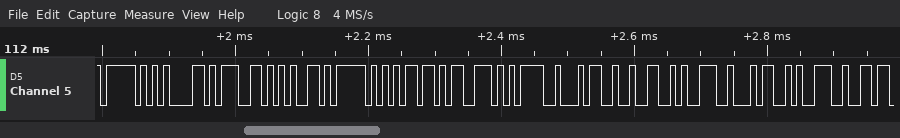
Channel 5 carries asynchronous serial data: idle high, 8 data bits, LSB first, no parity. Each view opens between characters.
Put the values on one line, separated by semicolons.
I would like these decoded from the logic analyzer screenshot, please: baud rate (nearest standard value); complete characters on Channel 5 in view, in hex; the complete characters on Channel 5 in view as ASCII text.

115200 baud; 5F, 61, 67, 65, 5F, 6D, 73, 3D, 34, 32, 39, 34, 39; "_age_ms=42949"
